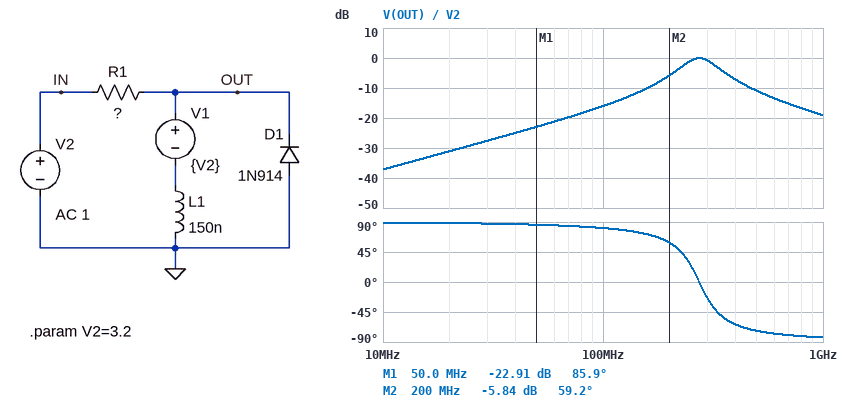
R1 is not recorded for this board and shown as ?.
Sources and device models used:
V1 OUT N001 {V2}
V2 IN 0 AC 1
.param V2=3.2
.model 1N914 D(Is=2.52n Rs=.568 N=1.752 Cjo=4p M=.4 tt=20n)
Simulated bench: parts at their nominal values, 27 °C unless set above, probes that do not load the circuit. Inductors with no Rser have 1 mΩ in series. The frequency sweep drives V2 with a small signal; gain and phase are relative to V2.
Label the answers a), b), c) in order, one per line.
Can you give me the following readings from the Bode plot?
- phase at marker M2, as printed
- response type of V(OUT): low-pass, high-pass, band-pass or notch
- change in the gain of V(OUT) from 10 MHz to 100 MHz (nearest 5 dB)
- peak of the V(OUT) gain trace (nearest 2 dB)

a) 59.2 deg
b) band-pass
c) 20 dB
d) 0 dB
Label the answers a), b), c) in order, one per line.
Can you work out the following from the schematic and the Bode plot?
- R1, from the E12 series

a) 680 Ω
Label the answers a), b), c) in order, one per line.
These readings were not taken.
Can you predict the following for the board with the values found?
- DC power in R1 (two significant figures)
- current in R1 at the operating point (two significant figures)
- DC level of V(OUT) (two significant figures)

a) 15 mW
b) 4.7 mA
c) 3.2 V
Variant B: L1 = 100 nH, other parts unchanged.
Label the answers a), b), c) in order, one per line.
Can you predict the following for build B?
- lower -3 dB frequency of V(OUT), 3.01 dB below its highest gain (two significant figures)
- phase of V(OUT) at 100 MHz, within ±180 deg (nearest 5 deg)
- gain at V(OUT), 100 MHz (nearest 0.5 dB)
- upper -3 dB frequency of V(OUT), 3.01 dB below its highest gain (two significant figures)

a) 290 MHz
b) 85 deg
c) -20.0 dB
d) 390 MHz
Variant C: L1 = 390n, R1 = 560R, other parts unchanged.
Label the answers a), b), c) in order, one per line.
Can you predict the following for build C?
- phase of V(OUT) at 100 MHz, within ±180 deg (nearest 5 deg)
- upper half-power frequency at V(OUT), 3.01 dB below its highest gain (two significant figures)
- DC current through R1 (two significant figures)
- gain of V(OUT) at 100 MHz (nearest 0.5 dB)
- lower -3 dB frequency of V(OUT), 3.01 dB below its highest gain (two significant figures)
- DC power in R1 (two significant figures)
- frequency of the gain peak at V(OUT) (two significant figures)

a) 55 deg
b) 240 MHz
c) 5.7 mA
d) -5.0 dB
e) 120 MHz
f) 18 mW
g) 170 MHz
